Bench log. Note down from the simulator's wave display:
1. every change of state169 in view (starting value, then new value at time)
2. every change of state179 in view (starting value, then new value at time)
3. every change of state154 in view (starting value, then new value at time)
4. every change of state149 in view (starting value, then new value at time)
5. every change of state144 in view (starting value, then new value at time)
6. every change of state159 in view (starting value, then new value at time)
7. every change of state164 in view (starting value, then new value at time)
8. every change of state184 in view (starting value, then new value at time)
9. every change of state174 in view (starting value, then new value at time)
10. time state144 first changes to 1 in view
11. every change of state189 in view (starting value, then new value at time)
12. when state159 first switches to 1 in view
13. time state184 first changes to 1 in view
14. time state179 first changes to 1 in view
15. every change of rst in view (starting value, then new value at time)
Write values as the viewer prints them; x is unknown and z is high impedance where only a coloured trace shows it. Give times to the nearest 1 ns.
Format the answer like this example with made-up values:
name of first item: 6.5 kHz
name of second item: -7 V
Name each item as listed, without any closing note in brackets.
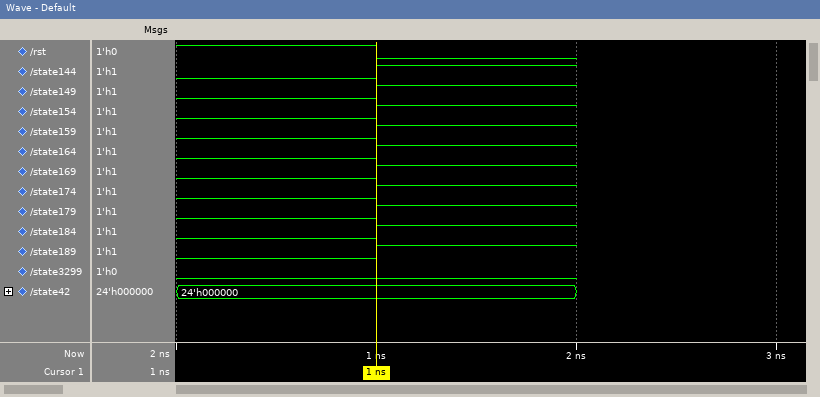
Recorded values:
every change of state169 in view: 0, 1 at 1 ns
every change of state179 in view: 0, 1 at 1 ns
every change of state154 in view: 0, 1 at 1 ns
every change of state149 in view: 0, 1 at 1 ns
every change of state144 in view: 0, 1 at 1 ns
every change of state159 in view: 0, 1 at 1 ns
every change of state164 in view: 0, 1 at 1 ns
every change of state184 in view: 0, 1 at 1 ns
every change of state174 in view: 0, 1 at 1 ns
time state144 first changes to 1 in view: 1 ns
every change of state189 in view: 0, 1 at 1 ns
when state159 first switches to 1 in view: 1 ns
time state184 first changes to 1 in view: 1 ns
time state179 first changes to 1 in view: 1 ns
every change of rst in view: 1, 0 at 1 ns
